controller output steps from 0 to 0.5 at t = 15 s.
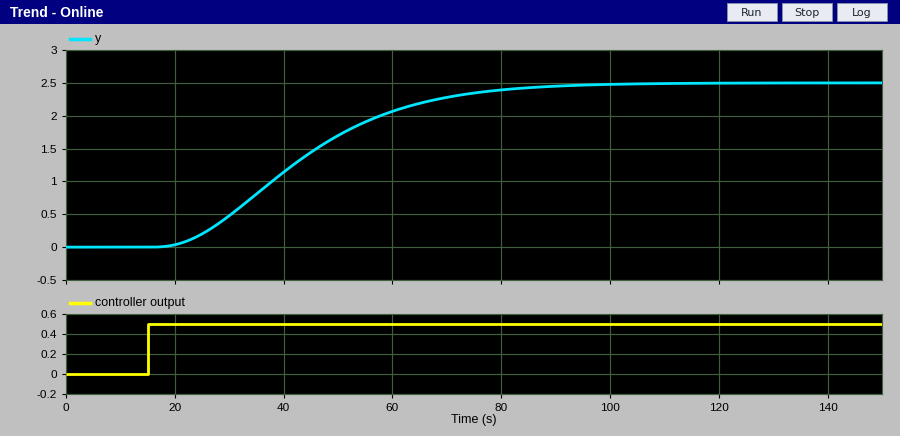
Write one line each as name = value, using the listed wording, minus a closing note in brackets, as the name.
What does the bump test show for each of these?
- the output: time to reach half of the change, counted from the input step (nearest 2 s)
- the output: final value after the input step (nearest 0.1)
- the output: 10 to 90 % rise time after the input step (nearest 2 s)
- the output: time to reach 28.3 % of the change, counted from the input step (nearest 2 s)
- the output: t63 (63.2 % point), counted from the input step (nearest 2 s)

the output: time to reach half of the change, counted from the input step = 26 s
the output: final value after the input step = 2.5
the output: 10 to 90 % rise time after the input step = 42 s
the output: time to reach 28.3 % of the change, counted from the input step = 18 s
the output: t63 (63.2 % point), counted from the input step = 32 s
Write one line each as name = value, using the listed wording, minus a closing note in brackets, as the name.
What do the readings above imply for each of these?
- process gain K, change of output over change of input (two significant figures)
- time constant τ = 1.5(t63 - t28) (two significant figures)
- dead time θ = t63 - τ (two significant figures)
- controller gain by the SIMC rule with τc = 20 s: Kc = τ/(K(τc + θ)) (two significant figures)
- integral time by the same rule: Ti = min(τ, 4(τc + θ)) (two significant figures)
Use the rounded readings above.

process gain K, change of output over change of input = 5.0
time constant τ = 1.5(t63 - t28) = 21 s
dead time θ = t63 - τ = 11 s
controller gain by the SIMC rule with τc = 20 s: Kc = τ/(K(τc + θ)) = 0.14
integral time by the same rule: Ti = min(τ, 4(τc + θ)) = 21 s
